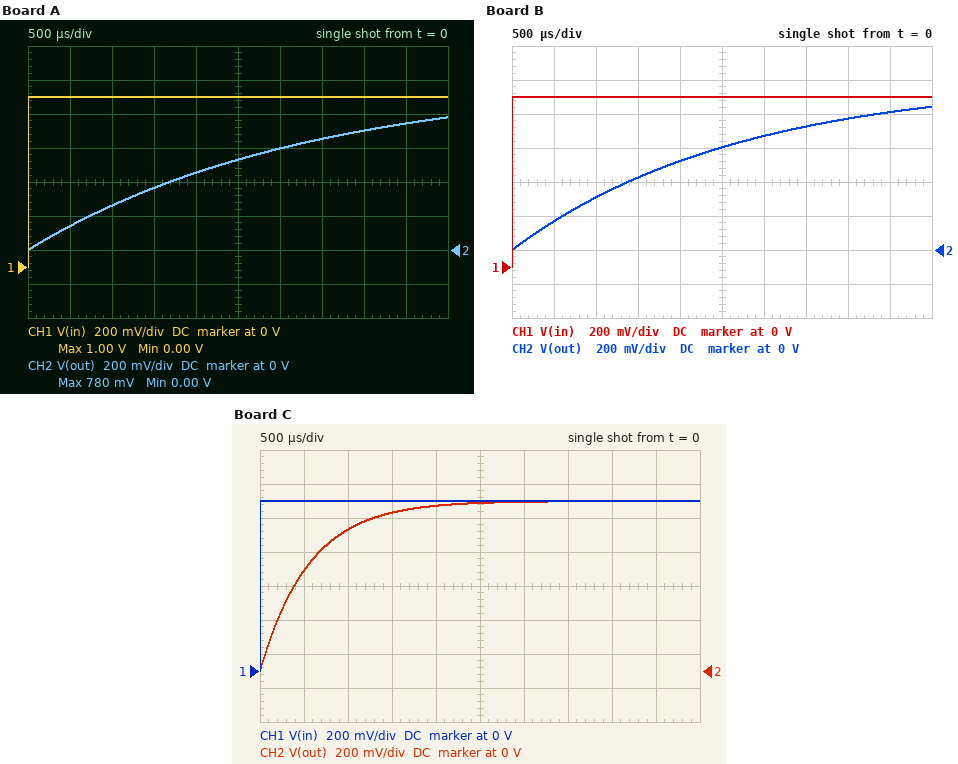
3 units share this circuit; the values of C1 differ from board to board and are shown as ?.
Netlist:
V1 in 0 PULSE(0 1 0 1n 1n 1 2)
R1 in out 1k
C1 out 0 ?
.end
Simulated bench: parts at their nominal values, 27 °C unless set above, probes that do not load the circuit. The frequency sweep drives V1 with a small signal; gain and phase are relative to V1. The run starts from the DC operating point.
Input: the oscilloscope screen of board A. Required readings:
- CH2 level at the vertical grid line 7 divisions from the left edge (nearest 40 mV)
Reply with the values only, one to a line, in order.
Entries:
640 mV
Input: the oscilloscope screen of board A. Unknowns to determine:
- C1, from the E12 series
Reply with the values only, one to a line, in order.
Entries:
3.3 µF
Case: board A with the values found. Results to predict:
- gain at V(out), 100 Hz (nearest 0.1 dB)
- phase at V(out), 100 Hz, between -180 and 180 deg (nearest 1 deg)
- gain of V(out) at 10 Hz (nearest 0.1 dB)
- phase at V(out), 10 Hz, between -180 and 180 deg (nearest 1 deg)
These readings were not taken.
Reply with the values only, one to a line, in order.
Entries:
-7.2 dB
-64 deg
-0.2 dB
-12 deg
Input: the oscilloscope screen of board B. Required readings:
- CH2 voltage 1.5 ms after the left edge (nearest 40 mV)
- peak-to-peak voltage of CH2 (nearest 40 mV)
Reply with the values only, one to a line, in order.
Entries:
440 mV
840 mV
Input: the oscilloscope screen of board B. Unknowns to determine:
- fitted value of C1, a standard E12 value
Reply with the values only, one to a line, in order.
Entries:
2.7 µF
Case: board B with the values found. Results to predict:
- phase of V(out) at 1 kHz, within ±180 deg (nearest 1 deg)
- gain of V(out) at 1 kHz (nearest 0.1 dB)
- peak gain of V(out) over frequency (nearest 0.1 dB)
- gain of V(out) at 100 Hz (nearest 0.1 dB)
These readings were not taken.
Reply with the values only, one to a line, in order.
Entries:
-87 deg
-24.6 dB
0 dB
-5.9 dB
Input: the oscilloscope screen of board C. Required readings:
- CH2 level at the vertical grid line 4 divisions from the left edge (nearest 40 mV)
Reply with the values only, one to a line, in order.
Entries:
960 mV
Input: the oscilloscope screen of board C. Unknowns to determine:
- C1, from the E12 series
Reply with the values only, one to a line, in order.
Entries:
560 nF
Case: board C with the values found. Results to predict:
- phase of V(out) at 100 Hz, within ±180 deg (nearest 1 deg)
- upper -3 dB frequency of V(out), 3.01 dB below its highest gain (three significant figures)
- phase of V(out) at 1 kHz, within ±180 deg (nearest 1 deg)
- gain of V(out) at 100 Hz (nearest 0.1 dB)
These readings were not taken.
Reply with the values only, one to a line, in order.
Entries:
-19 deg
284 Hz
-74 deg
-0.5 dB
